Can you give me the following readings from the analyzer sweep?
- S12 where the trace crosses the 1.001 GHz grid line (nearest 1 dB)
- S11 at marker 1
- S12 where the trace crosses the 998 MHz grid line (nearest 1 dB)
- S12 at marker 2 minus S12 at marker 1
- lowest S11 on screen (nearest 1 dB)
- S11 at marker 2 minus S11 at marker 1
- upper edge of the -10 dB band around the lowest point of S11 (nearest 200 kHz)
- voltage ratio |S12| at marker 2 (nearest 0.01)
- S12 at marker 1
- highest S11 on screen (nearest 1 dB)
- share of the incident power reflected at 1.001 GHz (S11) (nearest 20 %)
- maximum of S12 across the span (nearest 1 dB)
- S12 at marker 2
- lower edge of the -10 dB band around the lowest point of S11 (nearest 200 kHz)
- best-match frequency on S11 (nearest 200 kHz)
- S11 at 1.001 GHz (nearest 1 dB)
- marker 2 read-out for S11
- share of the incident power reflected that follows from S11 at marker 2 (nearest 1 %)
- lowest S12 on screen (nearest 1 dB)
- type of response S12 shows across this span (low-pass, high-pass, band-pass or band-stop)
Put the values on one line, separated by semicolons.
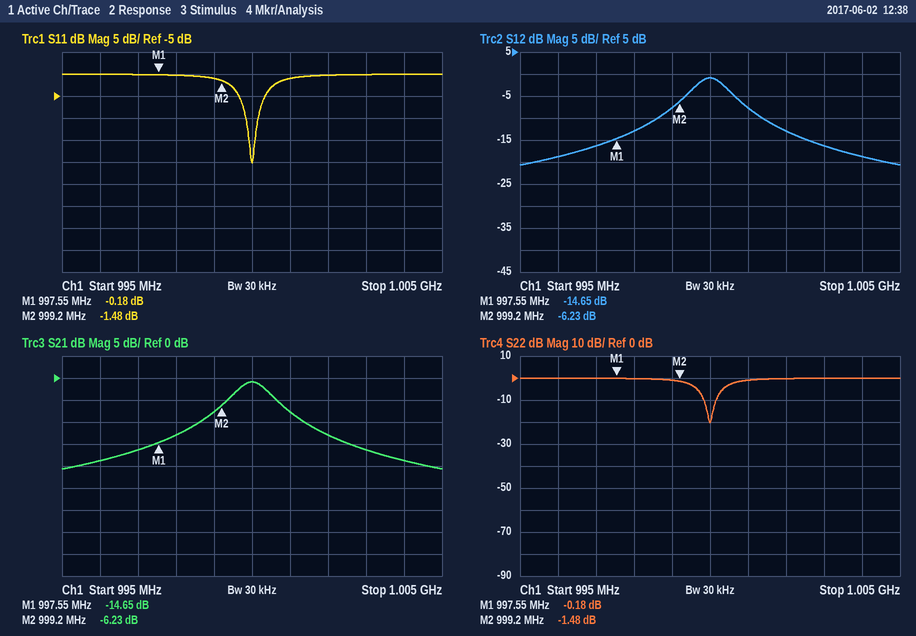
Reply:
-8 dB; -0.18 dB; -13 dB; 8.42 dB; -20 dB; -1.30 dB; 1.0002 GHz; 0.49; -14.65 dB; 0 dB; 80 %; -1 dB; -6.23 dB; 999.8 MHz; 1.0000 GHz; -1 dB; -1.48 dB; 71 %; -21 dB; band-pass
